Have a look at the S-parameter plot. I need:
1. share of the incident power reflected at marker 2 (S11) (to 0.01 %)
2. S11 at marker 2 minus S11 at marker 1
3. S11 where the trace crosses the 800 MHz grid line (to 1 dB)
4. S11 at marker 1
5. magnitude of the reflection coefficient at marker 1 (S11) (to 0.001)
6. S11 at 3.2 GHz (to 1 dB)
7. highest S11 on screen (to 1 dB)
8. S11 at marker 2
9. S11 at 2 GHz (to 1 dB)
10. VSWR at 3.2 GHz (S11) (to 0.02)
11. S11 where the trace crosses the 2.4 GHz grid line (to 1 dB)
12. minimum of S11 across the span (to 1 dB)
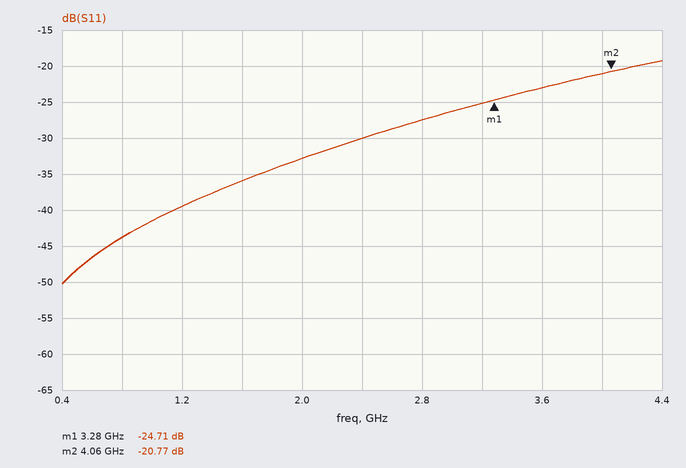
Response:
0.84 %
3.94 dB
-44 dB
-24.71 dB
0.058
-25 dB
-19 dB
-20.77 dB
-33 dB
1.12
-30 dB
-50 dB
